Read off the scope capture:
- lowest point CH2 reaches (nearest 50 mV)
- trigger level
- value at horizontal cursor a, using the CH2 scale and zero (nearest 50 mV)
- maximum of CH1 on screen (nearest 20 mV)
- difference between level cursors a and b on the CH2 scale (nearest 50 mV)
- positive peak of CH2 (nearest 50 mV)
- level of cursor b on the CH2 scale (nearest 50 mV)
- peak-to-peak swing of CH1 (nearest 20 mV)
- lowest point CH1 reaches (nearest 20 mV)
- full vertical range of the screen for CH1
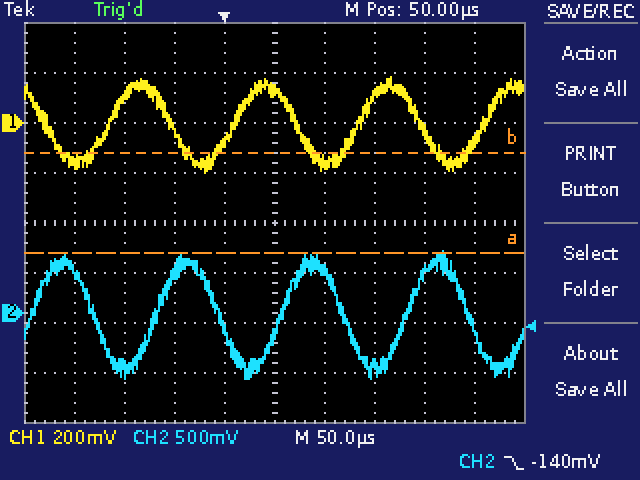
-650 mV
-140 mV
600 mV
180 mV
1.00 V
600 mV
1.60 V
380 mV
-200 mV
1.6 V
